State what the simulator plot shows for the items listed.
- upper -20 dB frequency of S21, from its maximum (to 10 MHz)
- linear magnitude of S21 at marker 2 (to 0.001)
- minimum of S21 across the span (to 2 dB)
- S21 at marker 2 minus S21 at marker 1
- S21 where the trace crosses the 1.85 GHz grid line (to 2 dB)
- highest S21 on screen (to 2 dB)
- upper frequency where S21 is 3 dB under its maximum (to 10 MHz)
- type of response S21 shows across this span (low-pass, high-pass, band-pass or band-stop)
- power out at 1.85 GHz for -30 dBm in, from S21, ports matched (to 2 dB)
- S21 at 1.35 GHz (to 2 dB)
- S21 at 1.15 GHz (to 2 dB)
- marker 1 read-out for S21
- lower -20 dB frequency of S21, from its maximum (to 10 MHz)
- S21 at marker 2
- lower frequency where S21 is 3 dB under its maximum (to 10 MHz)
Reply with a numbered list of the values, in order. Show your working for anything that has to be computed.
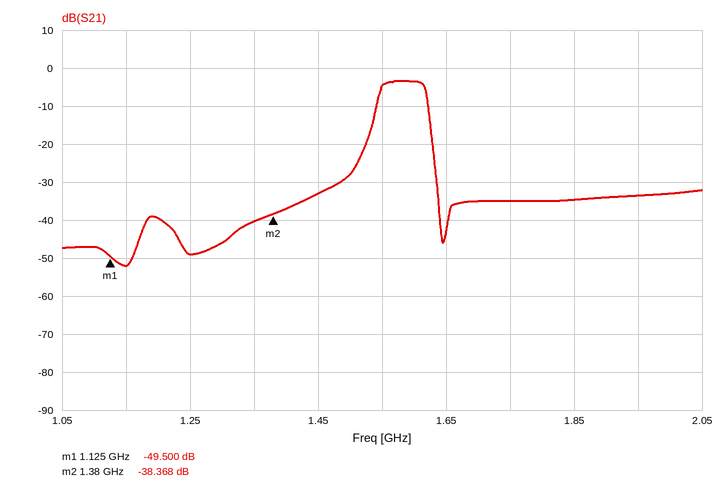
1. 1.63 GHz
2. 10^(-38.368/20) ≈ 0.012
3. -52 dB
4. -38.368 − (-49.5) = 11.132 dB
5. -34 dB
6. -4 dB
7. 1.62 GHz
8. band-pass
9. -30 dBm + (-34 dB) = -64 dBm
10. -40 dB
11. -52 dB
12. -49.500 dB
13. 1.52 GHz
14. -38.368 dB
15. 1.55 GHz
